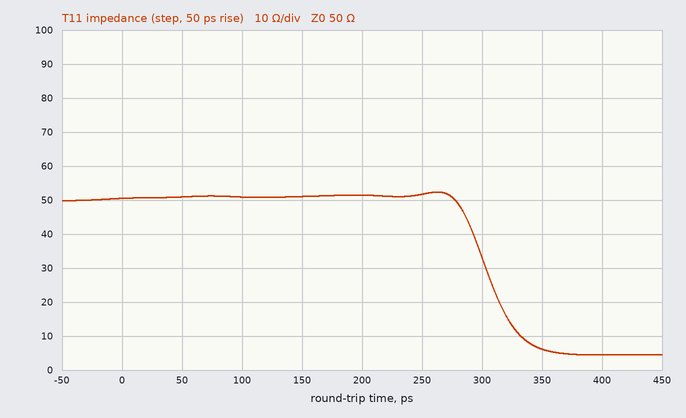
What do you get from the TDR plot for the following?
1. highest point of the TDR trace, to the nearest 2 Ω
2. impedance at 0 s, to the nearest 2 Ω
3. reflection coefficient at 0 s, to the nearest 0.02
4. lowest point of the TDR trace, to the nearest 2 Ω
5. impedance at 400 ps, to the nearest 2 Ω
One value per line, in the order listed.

52 Ω
50 Ω
0.00
4 Ω
4 Ω
